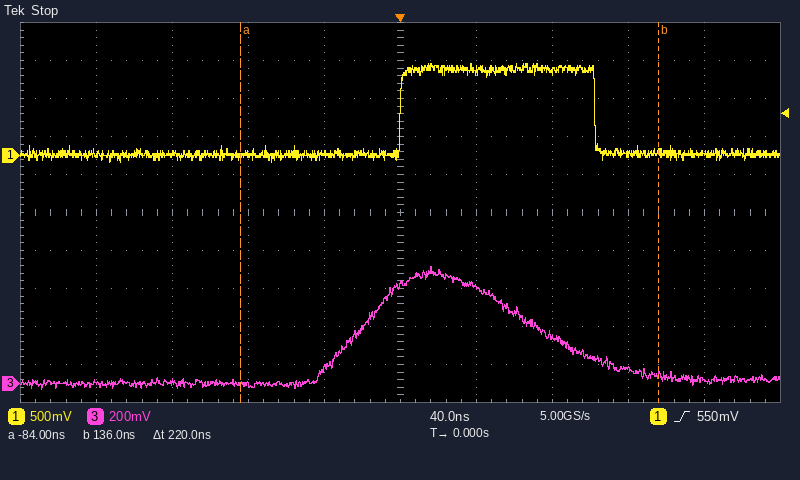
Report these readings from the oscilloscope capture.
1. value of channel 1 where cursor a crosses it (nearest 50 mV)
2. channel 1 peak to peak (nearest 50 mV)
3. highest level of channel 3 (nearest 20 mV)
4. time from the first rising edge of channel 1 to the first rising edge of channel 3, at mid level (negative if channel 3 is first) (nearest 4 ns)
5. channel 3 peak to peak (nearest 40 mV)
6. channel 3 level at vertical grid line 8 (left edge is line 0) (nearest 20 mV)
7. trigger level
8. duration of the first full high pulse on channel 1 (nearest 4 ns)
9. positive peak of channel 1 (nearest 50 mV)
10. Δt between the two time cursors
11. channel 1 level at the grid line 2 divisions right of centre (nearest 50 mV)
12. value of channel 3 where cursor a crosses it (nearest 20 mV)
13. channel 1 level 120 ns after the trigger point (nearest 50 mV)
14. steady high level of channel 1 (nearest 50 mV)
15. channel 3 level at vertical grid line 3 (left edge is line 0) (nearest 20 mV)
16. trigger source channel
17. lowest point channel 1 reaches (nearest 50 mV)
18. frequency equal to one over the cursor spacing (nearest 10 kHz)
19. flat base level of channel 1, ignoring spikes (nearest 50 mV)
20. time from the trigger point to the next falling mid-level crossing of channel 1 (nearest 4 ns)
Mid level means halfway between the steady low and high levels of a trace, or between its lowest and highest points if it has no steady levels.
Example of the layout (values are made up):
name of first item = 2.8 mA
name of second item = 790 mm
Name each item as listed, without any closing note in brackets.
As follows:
value of channel 1 where cursor a crosses it = 0 mV
channel 1 peak to peak = 1.30 V
highest level of channel 3 = 620 mV
time from the first rising edge of channel 1 to the first rising edge of channel 3, at mid level (negative if channel 3 is first) = -20 ns
channel 3 peak to peak = 640 mV
channel 3 level at vertical grid line 8 (left edge is line 0) = 80 mV
trigger level = 550 mV
duration of the first full high pulse on channel 1 = 104 ns
positive peak of channel 1 = 1.20 V
Δt between the two time cursors = 220 ns
channel 1 level at the grid line 2 divisions right of centre = 1.10 V
value of channel 3 where cursor a crosses it = 0 mV
channel 1 level 120 ns after the trigger point = 0 mV
steady high level of channel 1 = 1.15 V
channel 3 level at vertical grid line 3 (left edge is line 0) = 0 mV
trigger source channel = channel 1
lowest point channel 1 reaches = -100 mV
frequency equal to one over the cursor spacing = 4.55 MHz
flat base level of channel 1, ignoring spikes = 0 mV
time from the trigger point to the next falling mid-level crossing of channel 1 = 104 ns
